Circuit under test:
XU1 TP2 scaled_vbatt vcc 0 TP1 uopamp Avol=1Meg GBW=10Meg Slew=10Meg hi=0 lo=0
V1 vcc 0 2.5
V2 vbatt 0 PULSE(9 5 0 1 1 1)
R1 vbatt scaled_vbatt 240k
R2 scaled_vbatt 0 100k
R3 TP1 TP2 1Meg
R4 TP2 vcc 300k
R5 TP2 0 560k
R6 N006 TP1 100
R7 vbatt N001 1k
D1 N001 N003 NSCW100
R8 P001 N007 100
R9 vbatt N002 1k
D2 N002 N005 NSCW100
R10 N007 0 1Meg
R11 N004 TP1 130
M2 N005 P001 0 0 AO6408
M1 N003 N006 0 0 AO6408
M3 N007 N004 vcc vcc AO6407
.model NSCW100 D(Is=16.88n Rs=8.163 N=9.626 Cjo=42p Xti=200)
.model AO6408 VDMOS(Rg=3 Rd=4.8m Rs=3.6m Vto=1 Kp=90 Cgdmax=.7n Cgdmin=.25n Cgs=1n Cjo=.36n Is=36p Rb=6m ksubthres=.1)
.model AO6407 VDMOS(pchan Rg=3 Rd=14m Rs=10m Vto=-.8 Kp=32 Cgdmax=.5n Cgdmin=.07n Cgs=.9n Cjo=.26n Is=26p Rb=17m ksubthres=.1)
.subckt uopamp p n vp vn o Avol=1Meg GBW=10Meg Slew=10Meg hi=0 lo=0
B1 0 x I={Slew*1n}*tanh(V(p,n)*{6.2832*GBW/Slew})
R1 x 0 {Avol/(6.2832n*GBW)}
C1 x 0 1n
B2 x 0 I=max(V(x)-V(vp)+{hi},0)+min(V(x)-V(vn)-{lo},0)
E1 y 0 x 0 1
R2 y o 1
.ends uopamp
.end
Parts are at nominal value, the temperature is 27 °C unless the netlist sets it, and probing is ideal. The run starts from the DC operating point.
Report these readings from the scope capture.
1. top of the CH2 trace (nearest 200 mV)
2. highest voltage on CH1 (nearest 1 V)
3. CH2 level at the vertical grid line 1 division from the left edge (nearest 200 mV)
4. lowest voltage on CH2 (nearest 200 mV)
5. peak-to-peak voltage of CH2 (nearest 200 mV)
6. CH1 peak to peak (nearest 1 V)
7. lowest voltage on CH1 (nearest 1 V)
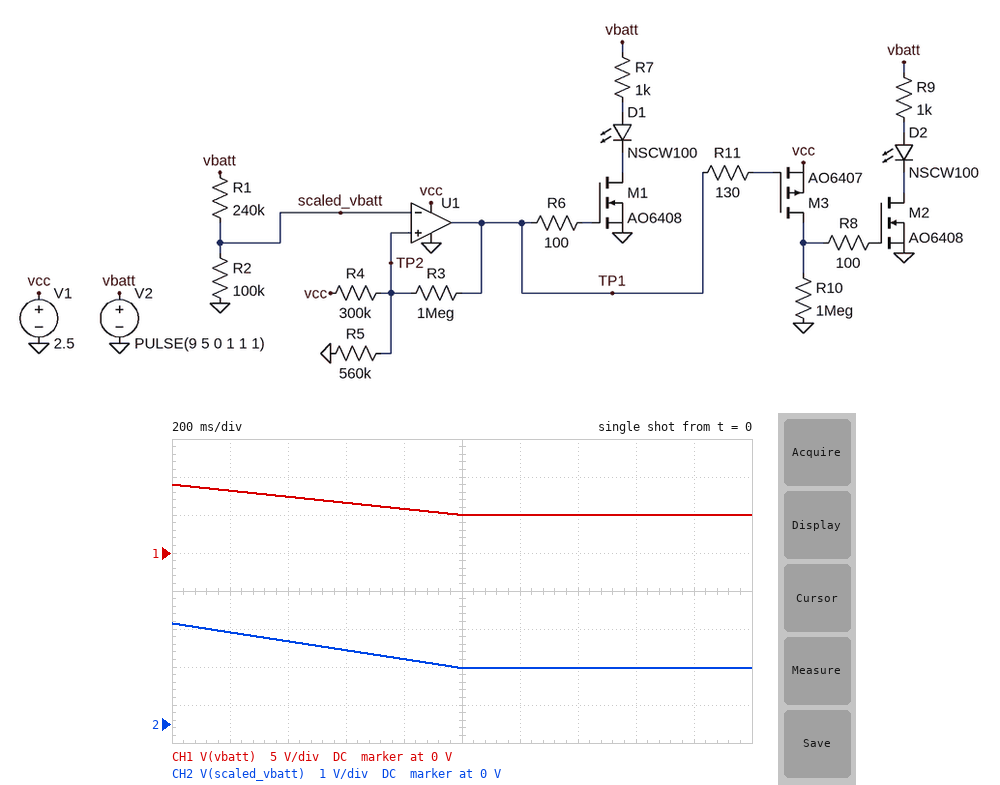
2.6 V
9 V
2.4 V
1.4 V
1.2 V
4 V
5 V
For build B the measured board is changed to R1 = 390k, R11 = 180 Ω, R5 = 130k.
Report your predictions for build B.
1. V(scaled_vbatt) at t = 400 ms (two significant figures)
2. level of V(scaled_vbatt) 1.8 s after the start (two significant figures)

1.5 V
1.0 V
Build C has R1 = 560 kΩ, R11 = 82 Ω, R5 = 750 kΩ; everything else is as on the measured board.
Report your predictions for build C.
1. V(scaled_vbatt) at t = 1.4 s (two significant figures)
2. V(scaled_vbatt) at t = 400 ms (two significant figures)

760 mV
1.1 V
